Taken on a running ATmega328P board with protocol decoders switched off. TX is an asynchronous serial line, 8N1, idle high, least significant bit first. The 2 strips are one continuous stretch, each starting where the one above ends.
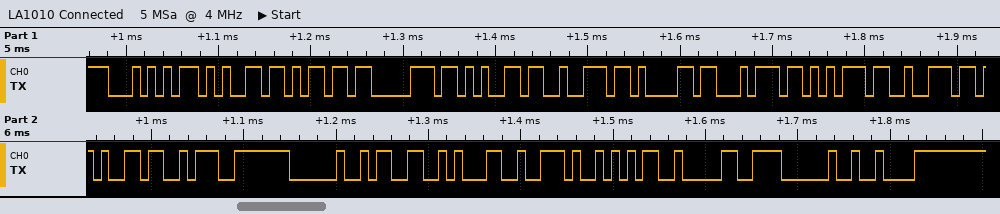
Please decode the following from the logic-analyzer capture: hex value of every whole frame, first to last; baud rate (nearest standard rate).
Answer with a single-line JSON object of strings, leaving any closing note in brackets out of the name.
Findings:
{"hex value of every whole frame, first to last": "54 65 6D 70 65 72 61 74 75 72 65 3A 20 33 31 2E 35 30 20 C2", "baud rate": "115200 baud"}
